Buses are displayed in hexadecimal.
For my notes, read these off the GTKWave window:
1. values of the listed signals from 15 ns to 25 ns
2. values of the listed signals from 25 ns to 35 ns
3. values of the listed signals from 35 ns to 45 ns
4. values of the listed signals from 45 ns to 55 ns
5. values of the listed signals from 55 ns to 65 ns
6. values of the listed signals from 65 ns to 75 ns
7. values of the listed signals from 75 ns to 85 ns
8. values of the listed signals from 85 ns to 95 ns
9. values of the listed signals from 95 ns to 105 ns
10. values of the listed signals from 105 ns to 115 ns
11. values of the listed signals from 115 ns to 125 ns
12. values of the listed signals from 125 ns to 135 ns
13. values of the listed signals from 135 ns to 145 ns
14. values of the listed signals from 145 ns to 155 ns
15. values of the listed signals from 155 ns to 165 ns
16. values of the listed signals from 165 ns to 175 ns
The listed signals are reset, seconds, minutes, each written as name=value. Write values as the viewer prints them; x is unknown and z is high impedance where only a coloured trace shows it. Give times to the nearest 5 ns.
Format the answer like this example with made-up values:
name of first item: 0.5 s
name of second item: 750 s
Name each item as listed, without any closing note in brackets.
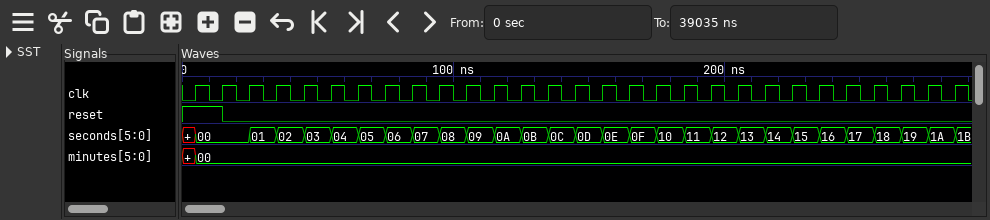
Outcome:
values of the listed signals from 15 ns to 25 ns: reset=0, seconds=00, minutes=00
values of the listed signals from 25 ns to 35 ns: reset=0, seconds=01, minutes=00
values of the listed signals from 35 ns to 45 ns: reset=0, seconds=02, minutes=00
values of the listed signals from 45 ns to 55 ns: reset=0, seconds=03, minutes=00
values of the listed signals from 55 ns to 65 ns: reset=0, seconds=04, minutes=00
values of the listed signals from 65 ns to 75 ns: reset=0, seconds=05, minutes=00
values of the listed signals from 75 ns to 85 ns: reset=0, seconds=06, minutes=00
values of the listed signals from 85 ns to 95 ns: reset=0, seconds=07, minutes=00
values of the listed signals from 95 ns to 105 ns: reset=0, seconds=08, minutes=00
values of the listed signals from 105 ns to 115 ns: reset=0, seconds=09, minutes=00
values of the listed signals from 115 ns to 125 ns: reset=0, seconds=0A, minutes=00
values of the listed signals from 125 ns to 135 ns: reset=0, seconds=0B, minutes=00
values of the listed signals from 135 ns to 145 ns: reset=0, seconds=0C, minutes=00
values of the listed signals from 145 ns to 155 ns: reset=0, seconds=0D, minutes=00
values of the listed signals from 155 ns to 165 ns: reset=0, seconds=0E, minutes=00
values of the listed signals from 165 ns to 175 ns: reset=0, seconds=0F, minutes=00
